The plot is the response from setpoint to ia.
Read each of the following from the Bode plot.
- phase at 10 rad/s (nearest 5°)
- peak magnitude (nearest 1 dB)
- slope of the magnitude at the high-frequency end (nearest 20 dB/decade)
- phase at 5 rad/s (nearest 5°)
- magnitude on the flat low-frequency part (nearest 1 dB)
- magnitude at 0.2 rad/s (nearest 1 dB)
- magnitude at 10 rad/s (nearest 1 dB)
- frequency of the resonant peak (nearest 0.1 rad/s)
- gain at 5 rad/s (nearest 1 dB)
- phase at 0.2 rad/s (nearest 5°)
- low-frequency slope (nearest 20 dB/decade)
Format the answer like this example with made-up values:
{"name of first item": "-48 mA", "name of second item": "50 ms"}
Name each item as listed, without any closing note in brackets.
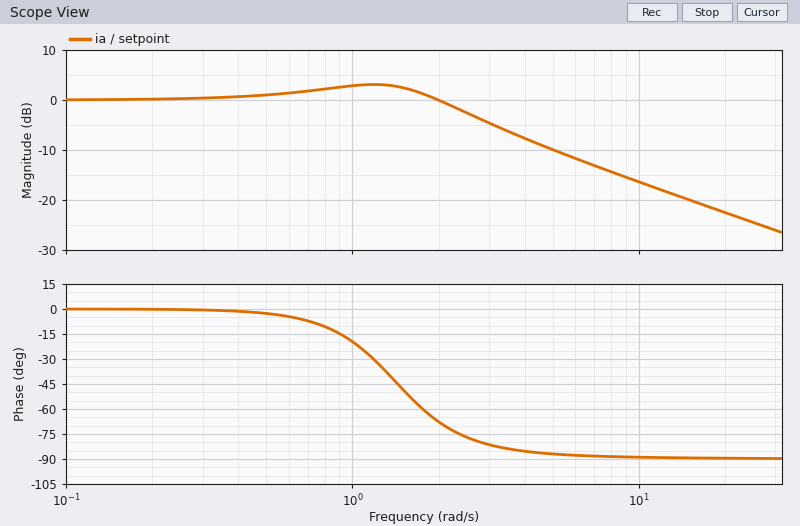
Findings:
{"phase at 10 rad/s": "-90°", "peak magnitude": "3 dB", "slope of the magnitude at the high-frequency end": "-20 dB/decade", "phase at 5 rad/s": "-85°", "magnitude on the flat low-frequency part": "0 dB", "magnitude at 0.2 rad/s": "0 dB", "magnitude at 10 rad/s": "-16 dB", "frequency of the resonant peak": "1.2 rad/s", "gain at 5 rad/s": "-10 dB", "phase at 0.2 rad/s": "0°", "low-frequency slope": "0 dB/decade"}
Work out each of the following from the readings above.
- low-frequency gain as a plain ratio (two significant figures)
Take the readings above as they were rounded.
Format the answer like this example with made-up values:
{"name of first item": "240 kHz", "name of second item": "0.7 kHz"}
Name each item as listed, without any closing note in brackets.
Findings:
{"low-frequency gain as a plain ratio": "1.0"}
